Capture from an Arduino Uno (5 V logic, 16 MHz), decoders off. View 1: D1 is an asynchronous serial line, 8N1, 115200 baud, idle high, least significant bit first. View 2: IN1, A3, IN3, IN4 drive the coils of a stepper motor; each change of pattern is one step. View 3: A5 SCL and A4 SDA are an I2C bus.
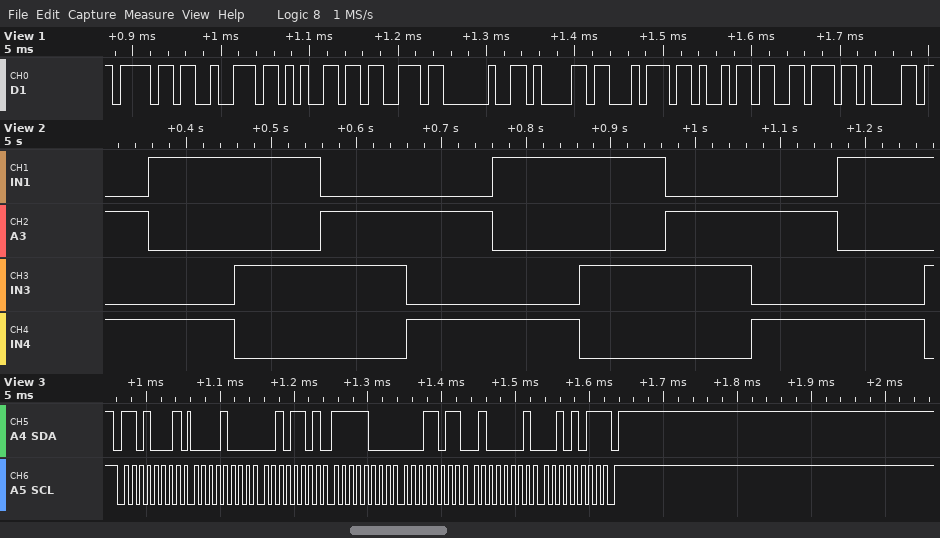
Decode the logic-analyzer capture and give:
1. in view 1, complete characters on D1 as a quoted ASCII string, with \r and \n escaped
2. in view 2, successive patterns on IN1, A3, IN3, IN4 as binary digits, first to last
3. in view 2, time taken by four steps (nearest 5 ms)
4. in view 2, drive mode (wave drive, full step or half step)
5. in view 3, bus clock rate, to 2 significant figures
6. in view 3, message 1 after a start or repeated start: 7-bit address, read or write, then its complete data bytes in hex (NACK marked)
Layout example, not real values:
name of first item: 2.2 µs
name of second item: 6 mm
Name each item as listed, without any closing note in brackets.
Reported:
in view 1, complete characters on D1 as a quoted ASCII string, with \r and \n escaped: "ores ativa"
in view 2, successive patterns on IN1, A3, IN3, IN4 as binary digits, first to last: 0101 1001 1010 0110 0101 1001 1010 0110 0101 1001 1010
in view 2, time taken by four steps: 405 ms
in view 2, drive mode: full step
in view 3, bus clock rate, to 2 significant figures: 100 kHz
in view 3, message 1 after a start or repeated start: 7-bit address, read or write, then its complete data bytes in hex: 0x68 read: 08 2D F8 1B 41 2B NACK
